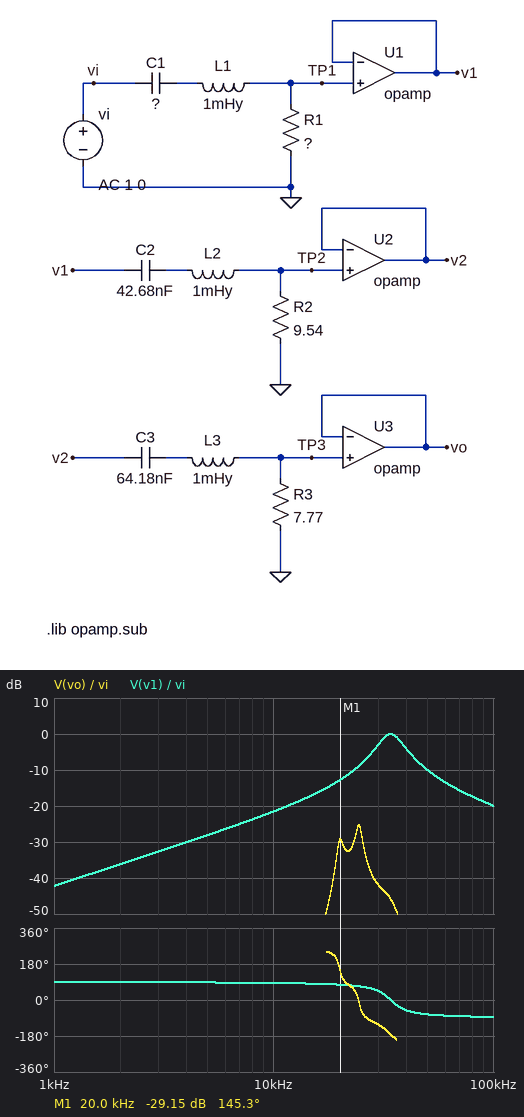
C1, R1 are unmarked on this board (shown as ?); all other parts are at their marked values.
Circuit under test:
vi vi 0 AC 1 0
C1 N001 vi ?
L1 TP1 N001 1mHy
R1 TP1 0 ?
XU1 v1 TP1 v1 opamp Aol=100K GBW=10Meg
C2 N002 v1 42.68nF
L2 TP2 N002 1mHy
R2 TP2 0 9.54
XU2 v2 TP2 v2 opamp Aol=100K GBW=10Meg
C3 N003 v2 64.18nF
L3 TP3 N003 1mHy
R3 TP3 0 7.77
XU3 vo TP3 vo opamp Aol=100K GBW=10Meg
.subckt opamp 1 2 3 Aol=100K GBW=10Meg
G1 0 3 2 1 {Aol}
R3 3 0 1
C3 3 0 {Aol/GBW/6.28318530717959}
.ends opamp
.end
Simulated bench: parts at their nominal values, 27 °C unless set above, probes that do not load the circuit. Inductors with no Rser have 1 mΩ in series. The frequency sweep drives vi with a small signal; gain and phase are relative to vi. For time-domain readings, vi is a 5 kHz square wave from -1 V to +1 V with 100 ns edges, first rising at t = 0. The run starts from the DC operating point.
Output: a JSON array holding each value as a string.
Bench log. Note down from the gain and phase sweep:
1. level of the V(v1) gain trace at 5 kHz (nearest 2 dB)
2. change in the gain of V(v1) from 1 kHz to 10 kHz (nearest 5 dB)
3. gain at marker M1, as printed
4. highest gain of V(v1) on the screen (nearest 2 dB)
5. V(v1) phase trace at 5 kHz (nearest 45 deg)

["-28 dB", "20 dB", "-29.15 dB", "0 dB", "90 deg"]
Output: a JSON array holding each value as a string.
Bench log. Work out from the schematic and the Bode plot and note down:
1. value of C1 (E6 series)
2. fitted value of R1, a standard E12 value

["22 nF", "56 Ω"]
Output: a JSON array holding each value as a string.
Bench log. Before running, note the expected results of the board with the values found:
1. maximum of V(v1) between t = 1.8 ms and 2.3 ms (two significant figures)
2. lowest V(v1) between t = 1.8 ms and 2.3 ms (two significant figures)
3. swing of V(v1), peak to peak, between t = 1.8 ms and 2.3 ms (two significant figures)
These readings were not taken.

["450 mV", "-450 mV", "900 mV"]
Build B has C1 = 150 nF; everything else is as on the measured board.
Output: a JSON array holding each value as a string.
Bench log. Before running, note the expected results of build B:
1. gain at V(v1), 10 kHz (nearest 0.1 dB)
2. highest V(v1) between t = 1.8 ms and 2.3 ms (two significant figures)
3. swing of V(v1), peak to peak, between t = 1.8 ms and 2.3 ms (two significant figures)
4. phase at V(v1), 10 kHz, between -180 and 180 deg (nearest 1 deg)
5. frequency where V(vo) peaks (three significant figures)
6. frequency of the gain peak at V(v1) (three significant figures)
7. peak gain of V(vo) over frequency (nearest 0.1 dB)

["-2.0 dB", "850 mV", "1.7 V", "38 deg", "19.9 kHz", "13.0 kHz", "-20.6 dB"]
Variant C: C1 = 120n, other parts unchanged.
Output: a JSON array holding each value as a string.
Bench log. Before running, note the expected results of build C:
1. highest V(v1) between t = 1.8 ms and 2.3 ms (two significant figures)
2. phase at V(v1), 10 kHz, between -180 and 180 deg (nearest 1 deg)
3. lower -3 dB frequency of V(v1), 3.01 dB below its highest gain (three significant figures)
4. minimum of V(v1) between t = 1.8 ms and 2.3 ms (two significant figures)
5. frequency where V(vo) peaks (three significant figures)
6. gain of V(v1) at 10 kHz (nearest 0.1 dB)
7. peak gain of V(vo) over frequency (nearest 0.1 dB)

["840 mV", "51 deg", "10.7 kHz", "-840 mV", "19.9 kHz", "-4.1 dB", "-19.6 dB"]
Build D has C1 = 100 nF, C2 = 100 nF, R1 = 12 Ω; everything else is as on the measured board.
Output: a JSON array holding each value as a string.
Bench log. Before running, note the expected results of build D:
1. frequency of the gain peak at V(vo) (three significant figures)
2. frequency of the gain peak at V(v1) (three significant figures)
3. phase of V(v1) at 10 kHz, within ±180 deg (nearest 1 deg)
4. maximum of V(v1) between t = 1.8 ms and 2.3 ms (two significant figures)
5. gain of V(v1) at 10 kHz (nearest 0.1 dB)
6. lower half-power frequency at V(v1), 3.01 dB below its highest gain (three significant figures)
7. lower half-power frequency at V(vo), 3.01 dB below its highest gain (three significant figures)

["16.0 kHz", "15.9 kHz", "83 deg", "370 mV", "-18.2 dB", "15.0 kHz", "15.5 kHz"]
